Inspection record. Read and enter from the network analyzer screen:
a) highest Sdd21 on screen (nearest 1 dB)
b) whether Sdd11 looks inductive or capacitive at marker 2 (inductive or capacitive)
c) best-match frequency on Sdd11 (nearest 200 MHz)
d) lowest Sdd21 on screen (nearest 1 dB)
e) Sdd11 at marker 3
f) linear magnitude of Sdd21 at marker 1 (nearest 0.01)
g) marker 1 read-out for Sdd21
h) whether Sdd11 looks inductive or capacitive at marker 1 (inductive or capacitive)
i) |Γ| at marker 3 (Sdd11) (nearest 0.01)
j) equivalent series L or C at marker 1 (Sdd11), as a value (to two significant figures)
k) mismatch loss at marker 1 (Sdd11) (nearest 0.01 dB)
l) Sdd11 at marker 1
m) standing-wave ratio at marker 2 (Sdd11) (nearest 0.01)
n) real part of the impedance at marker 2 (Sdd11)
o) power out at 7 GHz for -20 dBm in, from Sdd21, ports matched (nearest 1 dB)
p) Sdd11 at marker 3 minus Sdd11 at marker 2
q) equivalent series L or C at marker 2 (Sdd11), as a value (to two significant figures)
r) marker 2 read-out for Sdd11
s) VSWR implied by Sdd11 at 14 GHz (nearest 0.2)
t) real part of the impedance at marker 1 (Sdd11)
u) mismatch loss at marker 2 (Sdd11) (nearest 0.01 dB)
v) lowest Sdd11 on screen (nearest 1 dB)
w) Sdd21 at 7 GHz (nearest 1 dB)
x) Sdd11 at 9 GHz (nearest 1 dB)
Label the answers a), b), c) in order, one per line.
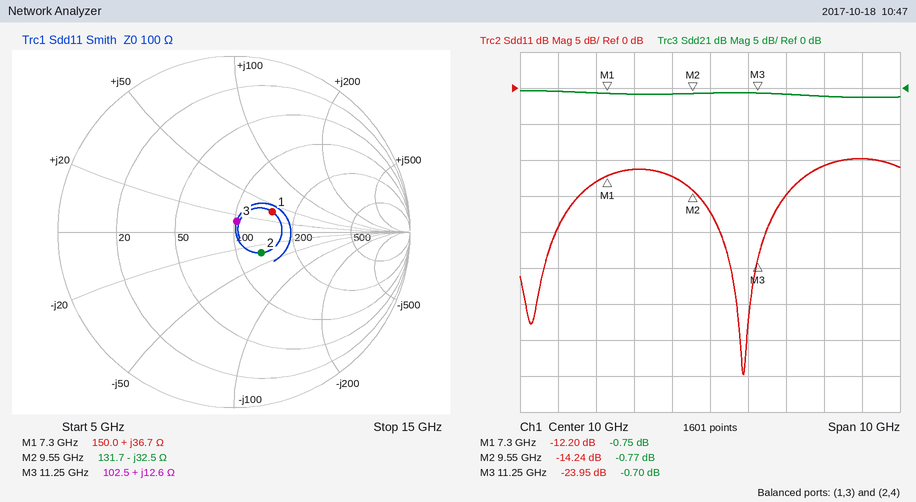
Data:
a) 0 dB
b) capacitive
c) 10.8 GHz
d) -1 dB
e) -23.95 dB
f) 0.92
g) -0.75 dB
h) inductive
i) 0.06
j) 800 pH
k) 0.27 dB
l) -12.20 dB
m) 1.48
n) 131.7 Ω
o) -21 dBm
p) -9.71 dB
q) 510 fF
r) -14.24 dB
s) 2.0
t) 150.0 Ω
u) 0.17 dB
v) -40 dB
w) -1 dB
x) -12 dB
